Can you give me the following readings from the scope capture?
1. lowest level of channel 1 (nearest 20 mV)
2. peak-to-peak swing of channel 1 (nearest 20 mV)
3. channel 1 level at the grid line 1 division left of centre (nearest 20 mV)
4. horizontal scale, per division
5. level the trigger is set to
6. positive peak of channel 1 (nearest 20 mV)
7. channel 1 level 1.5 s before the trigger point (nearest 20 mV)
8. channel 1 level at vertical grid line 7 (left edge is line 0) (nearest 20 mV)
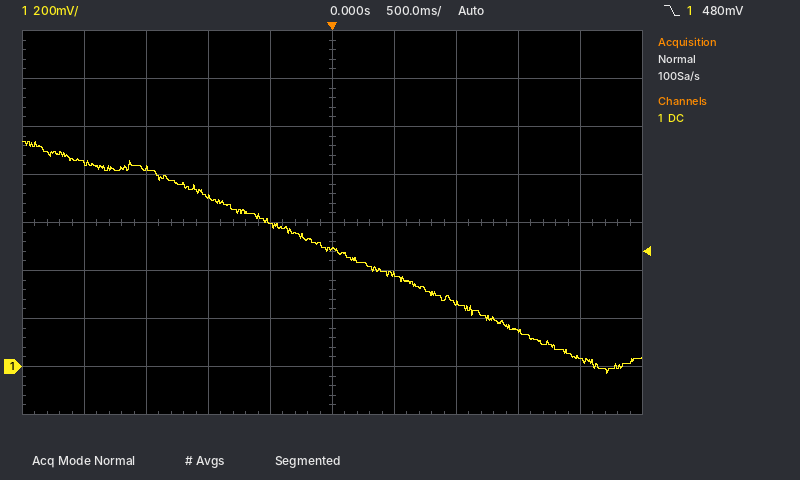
-20 mV
960 mV
600 mV
500 ms
480 mV
940 mV
820 mV
260 mV
